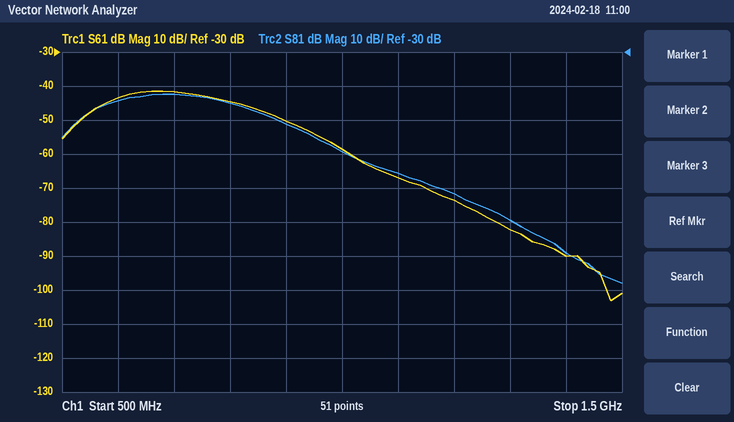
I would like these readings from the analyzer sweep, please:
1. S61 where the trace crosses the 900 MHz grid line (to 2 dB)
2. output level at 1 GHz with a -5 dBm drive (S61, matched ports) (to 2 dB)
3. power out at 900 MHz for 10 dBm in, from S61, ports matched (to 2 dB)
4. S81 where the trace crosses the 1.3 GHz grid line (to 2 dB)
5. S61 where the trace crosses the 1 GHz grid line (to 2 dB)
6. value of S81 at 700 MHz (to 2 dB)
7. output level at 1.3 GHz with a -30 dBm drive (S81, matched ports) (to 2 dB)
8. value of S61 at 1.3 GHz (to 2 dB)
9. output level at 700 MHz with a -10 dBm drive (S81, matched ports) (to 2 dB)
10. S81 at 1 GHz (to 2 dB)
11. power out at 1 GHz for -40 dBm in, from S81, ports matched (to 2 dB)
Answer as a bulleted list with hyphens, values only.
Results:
- -50 dB
- -64 dBm
- -40 dBm
- -80 dB
- -58 dB
- -42 dB
- -110 dBm
- -82 dB
- -52 dBm
- -60 dB
- -100 dBm
